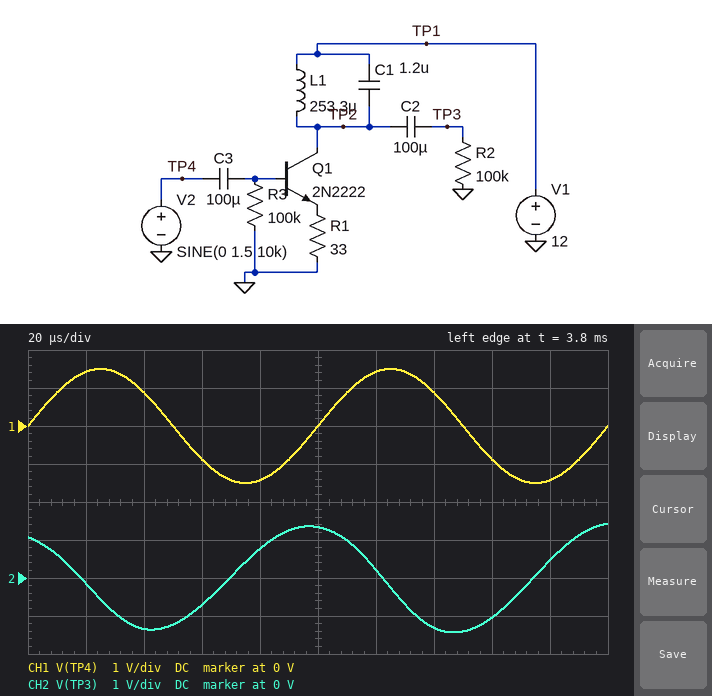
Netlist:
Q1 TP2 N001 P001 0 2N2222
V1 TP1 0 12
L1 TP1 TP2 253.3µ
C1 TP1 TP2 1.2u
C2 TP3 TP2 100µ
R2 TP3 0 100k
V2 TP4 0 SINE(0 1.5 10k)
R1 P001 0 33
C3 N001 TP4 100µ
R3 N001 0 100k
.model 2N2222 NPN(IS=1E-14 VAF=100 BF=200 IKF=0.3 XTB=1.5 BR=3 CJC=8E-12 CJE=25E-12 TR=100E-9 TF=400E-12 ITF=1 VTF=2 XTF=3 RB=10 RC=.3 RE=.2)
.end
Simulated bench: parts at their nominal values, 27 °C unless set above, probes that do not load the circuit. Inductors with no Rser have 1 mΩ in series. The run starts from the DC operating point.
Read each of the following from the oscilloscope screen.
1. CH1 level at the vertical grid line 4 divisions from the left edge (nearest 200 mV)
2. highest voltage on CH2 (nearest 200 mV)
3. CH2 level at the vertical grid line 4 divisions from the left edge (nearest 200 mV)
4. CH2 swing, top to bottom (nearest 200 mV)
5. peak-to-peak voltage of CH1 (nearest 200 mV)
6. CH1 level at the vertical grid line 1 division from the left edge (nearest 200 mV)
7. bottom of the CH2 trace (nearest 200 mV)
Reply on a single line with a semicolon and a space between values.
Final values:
-1.4 V; 1.4 V; 800 mV; 2.8 V; 3.0 V; 1.4 V; -1.4 V
